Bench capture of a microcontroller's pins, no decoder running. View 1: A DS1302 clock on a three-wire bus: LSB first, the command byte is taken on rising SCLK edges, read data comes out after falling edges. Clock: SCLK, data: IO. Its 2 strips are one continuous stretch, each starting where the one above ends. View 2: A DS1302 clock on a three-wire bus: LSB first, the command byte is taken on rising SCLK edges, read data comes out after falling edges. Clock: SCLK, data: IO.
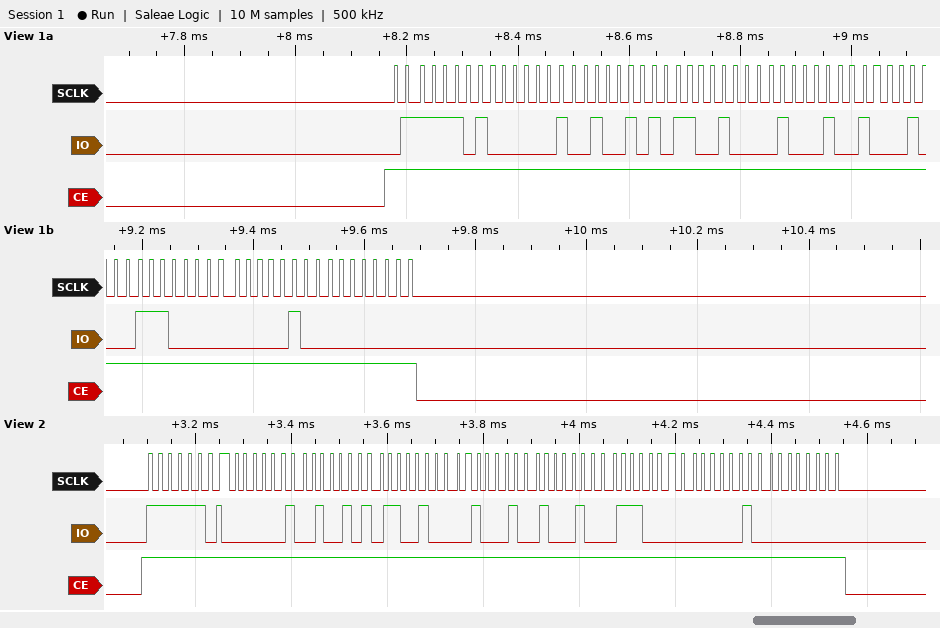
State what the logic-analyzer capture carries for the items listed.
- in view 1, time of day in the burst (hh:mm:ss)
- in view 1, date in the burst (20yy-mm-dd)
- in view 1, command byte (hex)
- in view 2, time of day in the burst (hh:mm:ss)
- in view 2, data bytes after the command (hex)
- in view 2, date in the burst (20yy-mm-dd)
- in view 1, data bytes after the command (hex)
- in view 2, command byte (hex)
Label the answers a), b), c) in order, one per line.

a) 13:52:40
b) 2020-11-22
c) 0xBE
d) 13:52:40
e) 40 52 13 22 11 07 20 00
f) 2020-11-22
g) 40 52 13 22 11 07 20 00
h) 0xBF
